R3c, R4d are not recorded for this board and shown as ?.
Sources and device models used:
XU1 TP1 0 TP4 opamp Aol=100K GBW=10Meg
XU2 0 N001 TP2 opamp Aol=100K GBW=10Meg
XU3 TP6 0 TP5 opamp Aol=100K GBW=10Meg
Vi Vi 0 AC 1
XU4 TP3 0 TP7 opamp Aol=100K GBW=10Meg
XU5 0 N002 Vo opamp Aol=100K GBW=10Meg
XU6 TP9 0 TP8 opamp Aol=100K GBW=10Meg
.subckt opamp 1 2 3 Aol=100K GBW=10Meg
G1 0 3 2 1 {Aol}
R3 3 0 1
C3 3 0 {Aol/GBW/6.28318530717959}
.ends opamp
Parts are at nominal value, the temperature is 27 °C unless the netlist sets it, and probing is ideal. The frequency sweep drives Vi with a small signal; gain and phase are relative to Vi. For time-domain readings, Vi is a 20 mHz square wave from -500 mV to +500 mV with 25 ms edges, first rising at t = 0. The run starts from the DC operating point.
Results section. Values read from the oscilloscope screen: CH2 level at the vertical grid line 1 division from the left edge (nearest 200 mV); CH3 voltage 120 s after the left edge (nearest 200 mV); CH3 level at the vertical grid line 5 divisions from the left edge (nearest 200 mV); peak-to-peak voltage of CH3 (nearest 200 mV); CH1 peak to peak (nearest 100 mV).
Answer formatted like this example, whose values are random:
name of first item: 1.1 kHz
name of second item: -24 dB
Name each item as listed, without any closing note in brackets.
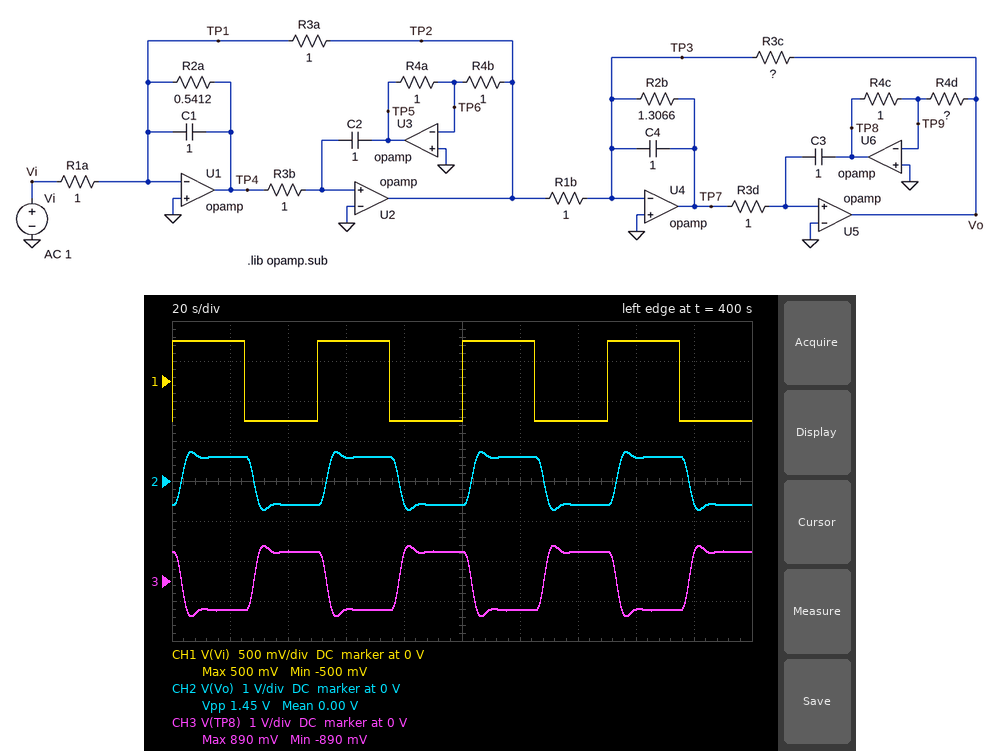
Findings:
CH2 level at the vertical grid line 1 division from the left edge: 600 mV
CH3 voltage 120 s after the left edge: -800 mV
CH3 level at the vertical grid line 5 divisions from the left edge: 800 mV
peak-to-peak voltage of CH3: 1.8 V
CH1 peak to peak: 1.0 V
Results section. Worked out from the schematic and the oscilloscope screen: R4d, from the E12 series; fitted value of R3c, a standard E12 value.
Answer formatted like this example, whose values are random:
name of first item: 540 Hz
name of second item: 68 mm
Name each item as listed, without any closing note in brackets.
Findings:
R4d, from the E12 series: 0.82 Ω
fitted value of R3c, a standard E12 value: 1.2 Ω
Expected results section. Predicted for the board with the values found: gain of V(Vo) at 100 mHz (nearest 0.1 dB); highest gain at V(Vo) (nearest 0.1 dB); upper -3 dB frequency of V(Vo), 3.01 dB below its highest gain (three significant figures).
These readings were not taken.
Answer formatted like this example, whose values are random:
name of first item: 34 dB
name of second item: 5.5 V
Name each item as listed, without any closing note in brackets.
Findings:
gain of V(Vo) at 100 mHz: 1.0 dB
highest gain at V(Vo): 1.7 dB
upper -3 dB frequency of V(Vo), 3.01 dB below its highest gain: 129 mHz
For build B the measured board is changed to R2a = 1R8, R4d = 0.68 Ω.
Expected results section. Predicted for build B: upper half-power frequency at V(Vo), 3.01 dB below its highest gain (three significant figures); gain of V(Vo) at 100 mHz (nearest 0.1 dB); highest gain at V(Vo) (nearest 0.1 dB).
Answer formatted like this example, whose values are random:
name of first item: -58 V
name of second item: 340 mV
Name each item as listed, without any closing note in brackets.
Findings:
upper half-power frequency at V(Vo), 3.01 dB below its highest gain: 159 mHz
gain of V(Vo) at 100 mHz: 5.6 dB
highest gain at V(Vo): 5.9 dB
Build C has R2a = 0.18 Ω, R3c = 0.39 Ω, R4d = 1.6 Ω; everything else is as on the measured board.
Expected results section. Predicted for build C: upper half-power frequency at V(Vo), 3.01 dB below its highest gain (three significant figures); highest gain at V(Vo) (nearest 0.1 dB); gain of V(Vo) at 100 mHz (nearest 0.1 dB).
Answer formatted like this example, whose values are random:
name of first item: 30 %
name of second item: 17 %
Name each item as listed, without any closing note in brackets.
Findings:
upper half-power frequency at V(Vo), 3.01 dB below its highest gain: 30.1 mHz
highest gain at V(Vo): -8.2 dB
gain of V(Vo) at 100 mHz: -18.4 dB
